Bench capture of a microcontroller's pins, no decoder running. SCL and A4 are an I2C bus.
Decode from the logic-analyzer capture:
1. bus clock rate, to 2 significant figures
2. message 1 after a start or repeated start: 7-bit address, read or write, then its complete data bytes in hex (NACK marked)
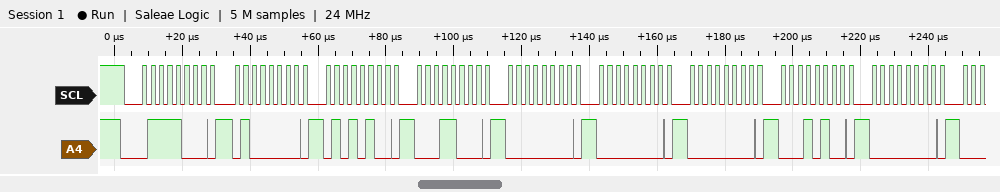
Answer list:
400 kHz
0x3C write: 40 54 18 00 00 00 14 00
